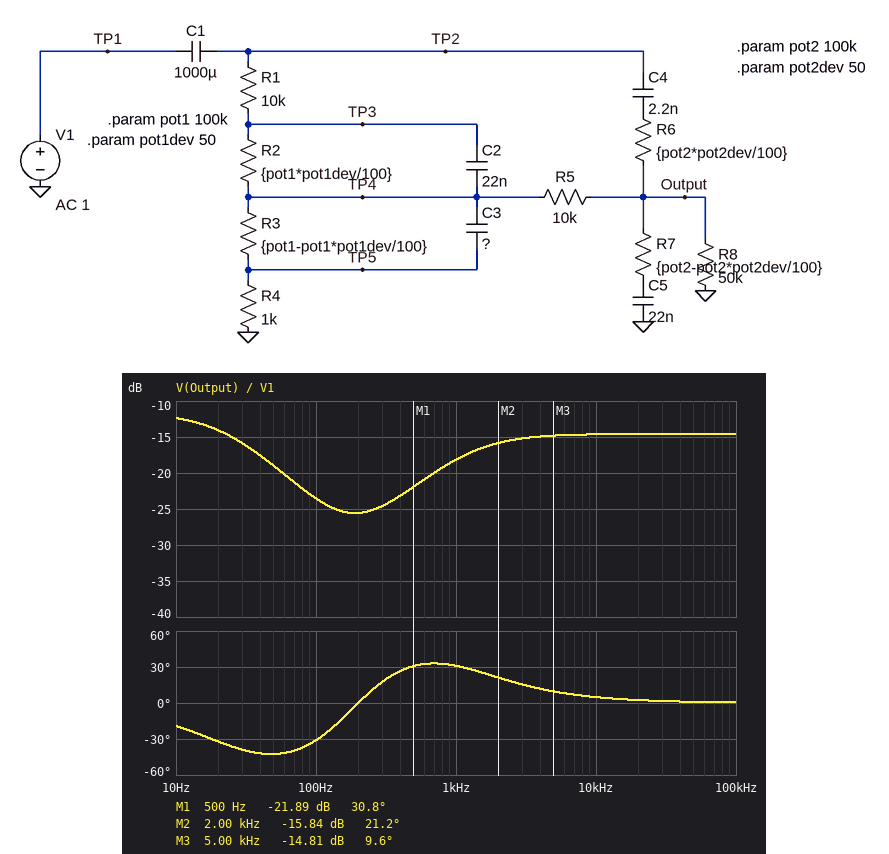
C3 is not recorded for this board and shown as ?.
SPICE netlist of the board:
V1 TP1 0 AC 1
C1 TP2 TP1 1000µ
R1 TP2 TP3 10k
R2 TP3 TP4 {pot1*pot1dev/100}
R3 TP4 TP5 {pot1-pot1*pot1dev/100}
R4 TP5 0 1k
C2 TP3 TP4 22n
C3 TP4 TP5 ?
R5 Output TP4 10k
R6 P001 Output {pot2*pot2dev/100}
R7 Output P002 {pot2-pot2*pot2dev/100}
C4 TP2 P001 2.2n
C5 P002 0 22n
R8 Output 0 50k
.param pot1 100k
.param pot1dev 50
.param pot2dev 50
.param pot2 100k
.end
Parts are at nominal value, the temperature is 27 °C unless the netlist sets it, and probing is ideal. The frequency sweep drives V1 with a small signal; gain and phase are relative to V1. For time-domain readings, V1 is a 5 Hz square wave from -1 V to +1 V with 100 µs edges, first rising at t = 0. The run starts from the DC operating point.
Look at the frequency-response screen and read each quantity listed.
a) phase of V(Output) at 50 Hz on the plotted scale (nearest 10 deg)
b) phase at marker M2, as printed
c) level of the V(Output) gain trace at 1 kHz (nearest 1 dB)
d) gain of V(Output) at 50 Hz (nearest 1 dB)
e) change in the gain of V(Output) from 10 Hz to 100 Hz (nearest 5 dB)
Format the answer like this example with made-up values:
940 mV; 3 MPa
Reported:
-40 deg; 21.2 deg; -18 dB; -19 dB; -10 dB
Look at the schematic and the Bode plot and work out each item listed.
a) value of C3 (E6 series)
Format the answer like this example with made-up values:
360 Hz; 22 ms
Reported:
330 nF
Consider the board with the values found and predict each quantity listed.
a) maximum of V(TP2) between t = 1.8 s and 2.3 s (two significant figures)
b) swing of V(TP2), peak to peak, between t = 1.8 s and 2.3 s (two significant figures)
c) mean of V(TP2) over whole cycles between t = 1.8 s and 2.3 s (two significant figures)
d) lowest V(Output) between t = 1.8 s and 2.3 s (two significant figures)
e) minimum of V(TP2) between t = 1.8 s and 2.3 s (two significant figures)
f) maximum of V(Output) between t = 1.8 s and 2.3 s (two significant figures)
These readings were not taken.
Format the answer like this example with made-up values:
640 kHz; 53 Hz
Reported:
2.0 V; 2.0 V; 980 mV; -6.5 mV; -25 mV; 520 mV
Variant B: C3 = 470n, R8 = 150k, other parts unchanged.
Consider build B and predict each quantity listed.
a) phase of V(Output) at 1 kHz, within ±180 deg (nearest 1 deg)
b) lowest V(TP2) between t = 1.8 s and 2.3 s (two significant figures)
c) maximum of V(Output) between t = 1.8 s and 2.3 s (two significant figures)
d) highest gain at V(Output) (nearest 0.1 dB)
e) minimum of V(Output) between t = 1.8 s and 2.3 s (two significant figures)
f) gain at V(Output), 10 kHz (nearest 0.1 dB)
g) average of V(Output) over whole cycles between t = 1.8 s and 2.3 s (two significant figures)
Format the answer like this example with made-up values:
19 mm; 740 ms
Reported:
33 deg; -22 mV; 730 mV; -8.7 dB; -7.9 mV; -13.8 dB; 360 mV
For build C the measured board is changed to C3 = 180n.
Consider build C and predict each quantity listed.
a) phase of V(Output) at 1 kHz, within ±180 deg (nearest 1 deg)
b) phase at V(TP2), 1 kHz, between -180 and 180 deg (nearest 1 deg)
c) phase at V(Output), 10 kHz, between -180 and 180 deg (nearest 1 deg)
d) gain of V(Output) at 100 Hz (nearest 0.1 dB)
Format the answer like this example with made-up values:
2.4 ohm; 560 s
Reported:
23 deg; 0 deg; 4 deg; -19.1 dB
